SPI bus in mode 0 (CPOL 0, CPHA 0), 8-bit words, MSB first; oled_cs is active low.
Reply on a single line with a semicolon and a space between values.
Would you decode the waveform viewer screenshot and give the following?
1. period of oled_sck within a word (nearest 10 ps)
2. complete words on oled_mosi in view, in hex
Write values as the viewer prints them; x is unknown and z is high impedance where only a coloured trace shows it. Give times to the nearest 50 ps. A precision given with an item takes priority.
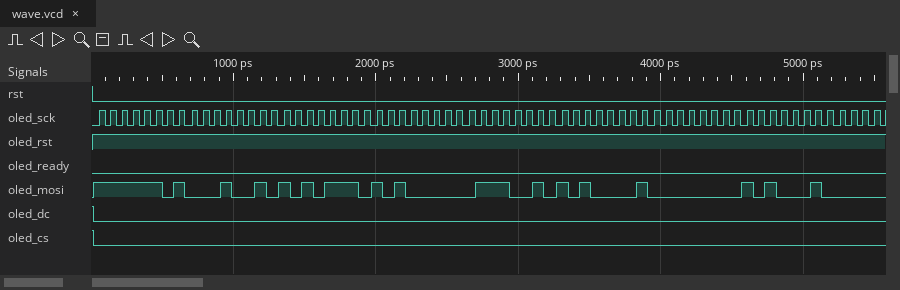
80 ps; FD, 12, AE, A0, 72, A1, 00, A2
